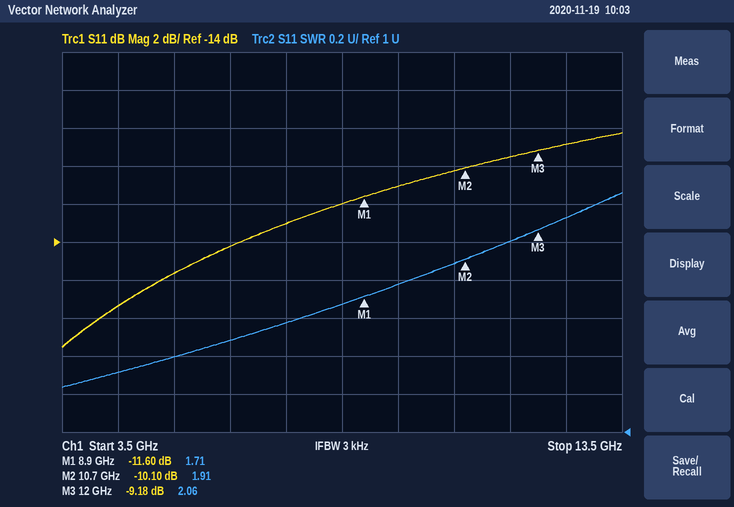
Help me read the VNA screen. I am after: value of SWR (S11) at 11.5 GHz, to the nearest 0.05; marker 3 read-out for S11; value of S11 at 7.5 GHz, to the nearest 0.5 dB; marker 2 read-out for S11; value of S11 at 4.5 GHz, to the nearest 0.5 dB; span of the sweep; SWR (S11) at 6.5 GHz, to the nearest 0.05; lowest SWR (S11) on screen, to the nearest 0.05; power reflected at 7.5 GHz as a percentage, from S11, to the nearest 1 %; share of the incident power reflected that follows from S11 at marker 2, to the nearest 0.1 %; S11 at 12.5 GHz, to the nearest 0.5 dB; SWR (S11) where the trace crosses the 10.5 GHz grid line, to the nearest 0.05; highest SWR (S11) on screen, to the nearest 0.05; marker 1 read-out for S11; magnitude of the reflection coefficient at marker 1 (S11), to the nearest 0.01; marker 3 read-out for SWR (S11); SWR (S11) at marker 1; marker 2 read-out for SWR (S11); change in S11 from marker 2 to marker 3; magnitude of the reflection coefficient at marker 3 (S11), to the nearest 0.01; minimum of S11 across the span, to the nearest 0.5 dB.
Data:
2.00
-9.18 dB
-13.0 dB
-10.10 dB
-17.5 dB
10 GHz
1.50
1.25
5 %
9.8 %
-9.0 dB
1.90
2.25
-11.60 dB
0.26
2.06
1.71
1.91
0.92 dB
0.35
-19.5 dB
